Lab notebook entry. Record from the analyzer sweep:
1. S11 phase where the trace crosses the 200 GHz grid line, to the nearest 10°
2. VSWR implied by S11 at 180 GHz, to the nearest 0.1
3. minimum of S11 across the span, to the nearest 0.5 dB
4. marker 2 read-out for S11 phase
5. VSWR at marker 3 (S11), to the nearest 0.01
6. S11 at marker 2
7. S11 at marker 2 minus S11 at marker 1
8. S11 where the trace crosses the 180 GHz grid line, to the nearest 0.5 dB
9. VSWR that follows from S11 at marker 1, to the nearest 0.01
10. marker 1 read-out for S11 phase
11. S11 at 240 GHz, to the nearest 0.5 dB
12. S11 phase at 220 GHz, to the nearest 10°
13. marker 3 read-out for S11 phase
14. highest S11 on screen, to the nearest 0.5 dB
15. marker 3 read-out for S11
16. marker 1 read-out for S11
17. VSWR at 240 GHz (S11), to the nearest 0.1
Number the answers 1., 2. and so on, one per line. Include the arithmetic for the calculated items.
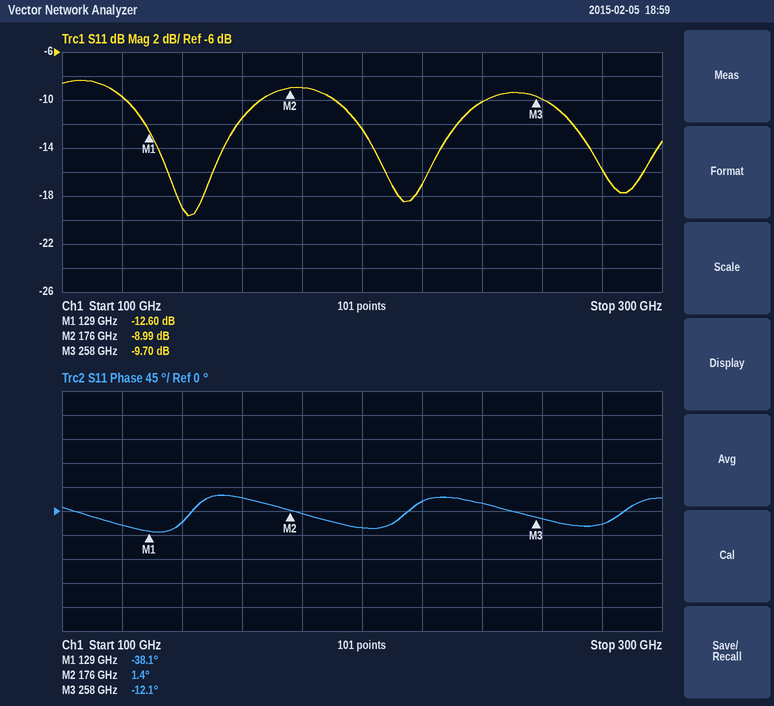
1. -30°
2. |Γ| = 10^(-9/20) = 0.3548; VSWR = (1 + 0.3548)/(1 − 0.3548) ≈ 2.1
3. -19.5 dB
4. 1.4°
5. (1 + 0.3273)/(1 − 0.3273) ≈ 1.97
6. -8.99 dB
7. -8.99 − (-12.6) = 3.61 dB
8. -9.0 dB
9. (1 + 0.2344)/(1 − 0.2344) ≈ 1.61
10. -38.1°
11. -10.0 dB
12. 20°
13. -12.1°
14. -8.5 dB
15. -9.70 dB
16. -12.60 dB
17. |Γ| = 10^(-10/20) = 0.3162; VSWR = (1 + 0.3162)/(1 − 0.3162) ≈ 1.9
